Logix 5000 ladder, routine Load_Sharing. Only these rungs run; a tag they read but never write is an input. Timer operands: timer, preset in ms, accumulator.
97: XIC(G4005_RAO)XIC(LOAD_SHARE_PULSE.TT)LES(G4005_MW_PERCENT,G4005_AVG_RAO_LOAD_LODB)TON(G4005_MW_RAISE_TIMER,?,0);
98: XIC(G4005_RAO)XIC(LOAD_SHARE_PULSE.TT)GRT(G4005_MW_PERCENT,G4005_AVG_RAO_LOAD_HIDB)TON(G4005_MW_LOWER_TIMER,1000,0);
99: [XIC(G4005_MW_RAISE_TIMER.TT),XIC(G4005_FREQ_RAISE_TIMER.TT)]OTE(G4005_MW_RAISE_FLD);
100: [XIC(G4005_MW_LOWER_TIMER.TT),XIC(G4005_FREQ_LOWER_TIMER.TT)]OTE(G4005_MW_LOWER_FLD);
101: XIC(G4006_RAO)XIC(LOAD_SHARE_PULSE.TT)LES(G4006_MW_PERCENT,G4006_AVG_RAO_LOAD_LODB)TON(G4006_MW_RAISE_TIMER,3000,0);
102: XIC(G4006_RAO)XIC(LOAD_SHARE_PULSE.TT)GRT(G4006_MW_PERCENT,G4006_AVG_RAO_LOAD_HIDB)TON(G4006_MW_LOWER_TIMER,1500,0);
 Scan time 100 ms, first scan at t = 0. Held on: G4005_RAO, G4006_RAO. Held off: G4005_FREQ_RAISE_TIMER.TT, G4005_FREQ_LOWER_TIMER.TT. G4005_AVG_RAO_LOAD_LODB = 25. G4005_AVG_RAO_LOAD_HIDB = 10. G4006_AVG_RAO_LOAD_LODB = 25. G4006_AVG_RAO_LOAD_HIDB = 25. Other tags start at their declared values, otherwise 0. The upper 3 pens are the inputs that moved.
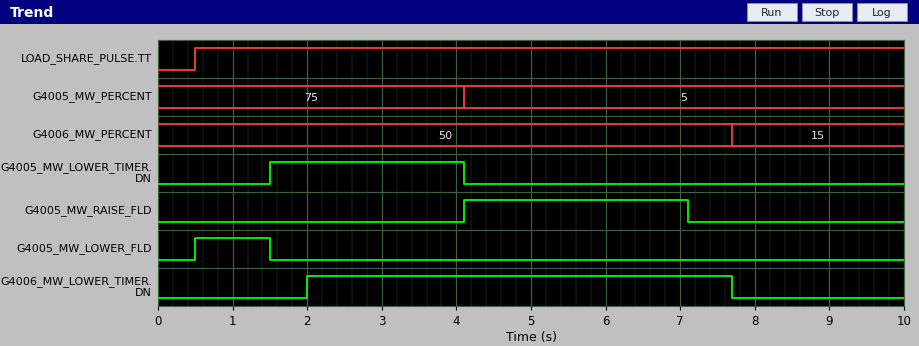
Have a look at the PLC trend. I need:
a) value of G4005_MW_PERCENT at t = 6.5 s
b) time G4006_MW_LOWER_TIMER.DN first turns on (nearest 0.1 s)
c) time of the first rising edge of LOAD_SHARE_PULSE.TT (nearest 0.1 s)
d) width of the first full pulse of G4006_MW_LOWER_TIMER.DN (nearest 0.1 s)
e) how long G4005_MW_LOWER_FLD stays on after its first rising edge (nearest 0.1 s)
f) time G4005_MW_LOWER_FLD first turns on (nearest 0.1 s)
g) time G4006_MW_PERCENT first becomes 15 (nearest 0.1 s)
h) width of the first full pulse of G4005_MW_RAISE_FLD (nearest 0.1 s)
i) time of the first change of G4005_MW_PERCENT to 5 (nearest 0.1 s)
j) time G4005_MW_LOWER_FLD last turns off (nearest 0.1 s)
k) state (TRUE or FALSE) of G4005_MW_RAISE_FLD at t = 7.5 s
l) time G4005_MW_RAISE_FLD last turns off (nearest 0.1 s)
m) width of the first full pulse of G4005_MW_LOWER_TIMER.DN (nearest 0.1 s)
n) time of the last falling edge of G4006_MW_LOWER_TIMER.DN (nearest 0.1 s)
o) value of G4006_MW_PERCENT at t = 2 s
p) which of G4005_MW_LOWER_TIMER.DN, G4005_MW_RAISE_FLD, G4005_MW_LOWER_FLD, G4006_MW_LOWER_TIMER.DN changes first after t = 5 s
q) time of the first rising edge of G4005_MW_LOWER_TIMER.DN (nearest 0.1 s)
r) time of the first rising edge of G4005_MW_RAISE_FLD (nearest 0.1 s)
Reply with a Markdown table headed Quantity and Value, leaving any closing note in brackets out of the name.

| Quantity | Value |
|---|---|
| value of G4005_MW_PERCENT at t = 6.5 s | 5 |
| time G4006_MW_LOWER_TIMER.DN first turns on | 2.0 s |
| time of the first rising edge of LOAD_SHARE_PULSE.TT | 0.5 s |
| width of the first full pulse of G4006_MW_LOWER_TIMER.DN | 5.7 s |
| how long G4005_MW_LOWER_FLD stays on after its first rising edge | 1.0 s |
| time G4005_MW_LOWER_FLD first turns on | 0.5 s |
| time G4006_MW_PERCENT first becomes 15 | 7.7 s |
| width of the first full pulse of G4005_MW_RAISE_FLD | 3.0 s |
| time of the first change of G4005_MW_PERCENT to 5 | 4.1 s |
| time G4005_MW_LOWER_FLD last turns off | 1.5 s |
| state (TRUE or FALSE) of G4005_MW_RAISE_FLD at t = 7.5 s | FALSE |
| time G4005_MW_RAISE_FLD last turns off | 7.1 s |
| width of the first full pulse of G4005_MW_LOWER_TIMER.DN | 2.6 s |
| time of the last falling edge of G4006_MW_LOWER_TIMER.DN | 7.7 s |
| value of G4006_MW_PERCENT at t = 2 s | 50 |
| which of G4005_MW_LOWER_TIMER.DN, G4005_MW_RAISE_FLD, G4005_MW_LOWER_FLD, G4006_MW_LOWER_TIMER.DN changes first after t = 5 s | G4005_MW_RAISE_FLD |
| time of the first rising edge of G4005_MW_LOWER_TIMER.DN | 1.5 s |
| time of the first rising edge of G4005_MW_RAISE_FLD | 4.1 s |
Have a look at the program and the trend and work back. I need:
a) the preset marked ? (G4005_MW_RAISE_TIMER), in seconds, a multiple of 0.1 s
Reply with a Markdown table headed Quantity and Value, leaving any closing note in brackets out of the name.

| Quantity | Value |
|---|---|
| the preset marked ? (G4005_MW_RAISE_TIMER), in seconds, a multiple of 0.1 s | 3.0 s |
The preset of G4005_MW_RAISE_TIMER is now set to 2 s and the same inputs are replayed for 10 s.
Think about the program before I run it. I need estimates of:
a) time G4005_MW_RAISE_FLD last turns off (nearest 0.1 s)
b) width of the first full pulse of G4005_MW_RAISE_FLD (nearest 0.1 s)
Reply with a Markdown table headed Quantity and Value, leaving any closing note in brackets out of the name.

| Quantity | Value |
|---|---|
| time G4005_MW_RAISE_FLD last turns off | 6.1 s |
| width of the first full pulse of G4005_MW_RAISE_FLD | 2.0 s |
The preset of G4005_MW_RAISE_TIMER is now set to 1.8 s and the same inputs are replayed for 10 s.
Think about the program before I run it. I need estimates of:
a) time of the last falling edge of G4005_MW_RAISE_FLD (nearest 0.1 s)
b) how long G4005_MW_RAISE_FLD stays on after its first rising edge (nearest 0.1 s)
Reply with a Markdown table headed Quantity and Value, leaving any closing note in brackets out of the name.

| Quantity | Value |
|---|---|
| time of the last falling edge of G4005_MW_RAISE_FLD | 5.9 s |
| how long G4005_MW_RAISE_FLD stays on after its first rising edge | 1.8 s |
